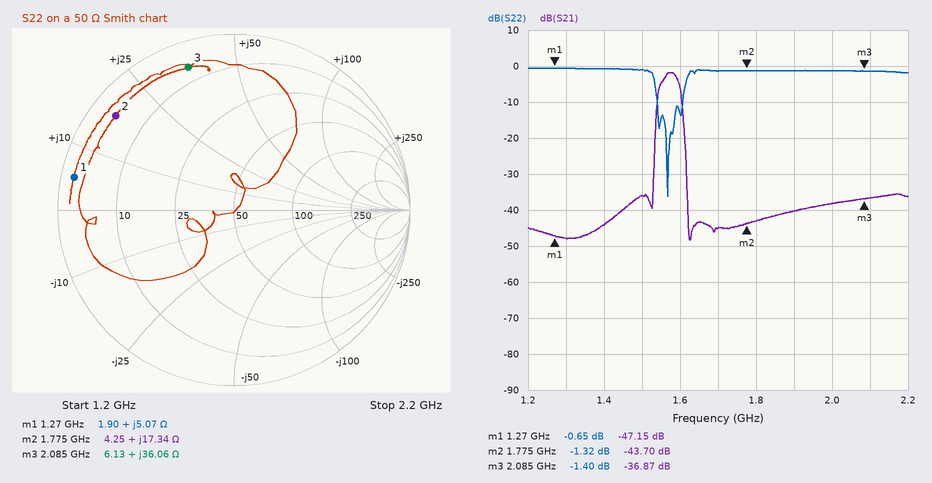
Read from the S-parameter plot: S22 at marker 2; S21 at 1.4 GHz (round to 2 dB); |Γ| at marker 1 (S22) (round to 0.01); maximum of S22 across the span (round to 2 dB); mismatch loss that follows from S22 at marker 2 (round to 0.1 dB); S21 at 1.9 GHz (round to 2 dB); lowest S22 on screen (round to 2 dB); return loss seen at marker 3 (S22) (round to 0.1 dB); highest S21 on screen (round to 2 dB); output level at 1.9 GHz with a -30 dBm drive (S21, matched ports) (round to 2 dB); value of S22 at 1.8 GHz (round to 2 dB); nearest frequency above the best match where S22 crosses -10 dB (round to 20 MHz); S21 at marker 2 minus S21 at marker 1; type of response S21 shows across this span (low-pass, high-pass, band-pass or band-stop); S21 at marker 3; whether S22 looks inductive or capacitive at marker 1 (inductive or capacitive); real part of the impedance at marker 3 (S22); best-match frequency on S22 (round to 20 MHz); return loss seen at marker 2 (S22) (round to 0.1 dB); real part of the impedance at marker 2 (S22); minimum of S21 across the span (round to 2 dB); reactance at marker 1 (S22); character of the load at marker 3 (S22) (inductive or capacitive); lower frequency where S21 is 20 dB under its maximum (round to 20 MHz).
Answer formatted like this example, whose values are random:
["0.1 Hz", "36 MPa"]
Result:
["-1.32 dB", "-44 dB", "0.93", "0 dB", "5.8 dB", "-40 dB", "-36 dB", "1.4 dB", "-2 dB", "-70 dBm", "-2 dB", "1.60 GHz", "3.45 dB", "band-pass", "-36.87 dB", "inductive", "6.13 Ω", "1.56 GHz", "1.3 dB", "4.25 Ω", "-48 dB", "+5.07 Ω", "inductive", "1.54 GHz"]
